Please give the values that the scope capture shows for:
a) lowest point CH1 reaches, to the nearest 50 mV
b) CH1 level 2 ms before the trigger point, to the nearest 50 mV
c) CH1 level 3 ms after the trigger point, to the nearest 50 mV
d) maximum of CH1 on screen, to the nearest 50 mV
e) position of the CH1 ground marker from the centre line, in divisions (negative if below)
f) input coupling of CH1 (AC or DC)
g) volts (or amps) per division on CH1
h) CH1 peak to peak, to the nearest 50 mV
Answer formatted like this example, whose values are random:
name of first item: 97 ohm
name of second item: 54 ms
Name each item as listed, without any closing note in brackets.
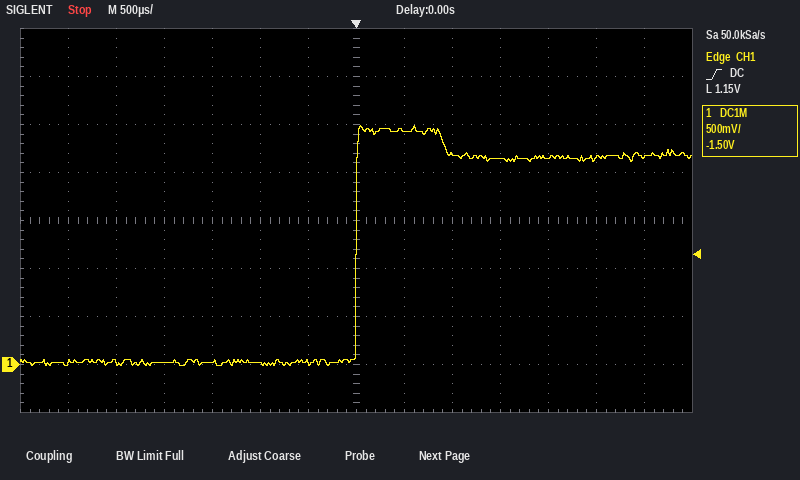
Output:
lowest point CH1 reaches, to the nearest 50 mV: 0 mV
CH1 level 2 ms before the trigger point, to the nearest 50 mV: 0 mV
CH1 level 3 ms after the trigger point, to the nearest 50 mV: 2.15 V
maximum of CH1 on screen, to the nearest 50 mV: 2.50 V
position of the CH1 ground marker from the centre line, in divisions: -3.0 div
input coupling of CH1: DC
volts (or amps) per division on CH1: 500 mV
CH1 peak to peak, to the nearest 50 mV: 2.50 V
